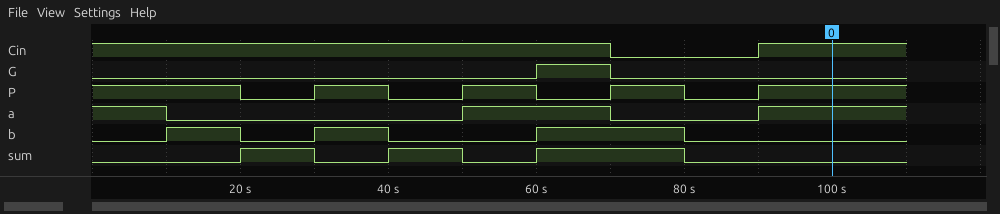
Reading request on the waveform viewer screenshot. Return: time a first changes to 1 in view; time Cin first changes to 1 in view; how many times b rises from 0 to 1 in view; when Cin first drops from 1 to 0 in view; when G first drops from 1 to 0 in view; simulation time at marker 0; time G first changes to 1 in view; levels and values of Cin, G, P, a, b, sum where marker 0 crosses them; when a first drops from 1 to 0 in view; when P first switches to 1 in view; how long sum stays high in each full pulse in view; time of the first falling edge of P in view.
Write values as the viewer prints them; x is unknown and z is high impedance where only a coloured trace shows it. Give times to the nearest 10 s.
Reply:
50 s
90 s
3
70 s
70 s
100 s
60 s
Cin=1, G=0, P=1, a=1, b=0, sum=0
10 s
30 s
10 s, 10 s, 20 s
20 s
